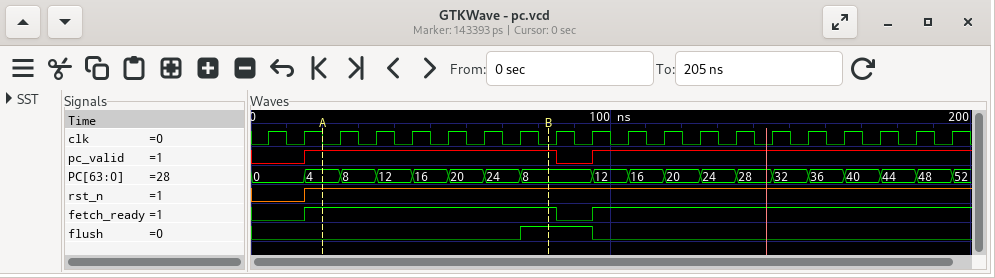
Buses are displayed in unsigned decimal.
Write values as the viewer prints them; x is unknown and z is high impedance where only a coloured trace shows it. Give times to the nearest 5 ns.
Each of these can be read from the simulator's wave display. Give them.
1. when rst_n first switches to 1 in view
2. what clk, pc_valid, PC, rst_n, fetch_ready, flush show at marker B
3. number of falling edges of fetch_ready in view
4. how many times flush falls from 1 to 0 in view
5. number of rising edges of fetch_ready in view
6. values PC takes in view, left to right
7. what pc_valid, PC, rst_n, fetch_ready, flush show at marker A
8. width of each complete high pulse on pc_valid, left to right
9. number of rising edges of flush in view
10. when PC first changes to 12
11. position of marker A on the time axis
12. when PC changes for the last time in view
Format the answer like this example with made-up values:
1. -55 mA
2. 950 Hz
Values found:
1. 15 ns
2. clk=0, pc_valid=1, PC=8, rst_n=1, fetch_ready=1, flush=1
3. 1
4. 1
5. 2
6. 0, 4, 8, 12, 16, 20, 24, 8, 12, 16, 20, 24, 28, 32, 36, 40, 44, 48, 52
7. pc_valid=1, PC=4, rst_n=1, fetch_ready=1, flush=0
8. 70 ns
9. 1
10. 35 ns
11. 20 ns
12. 195 ns
